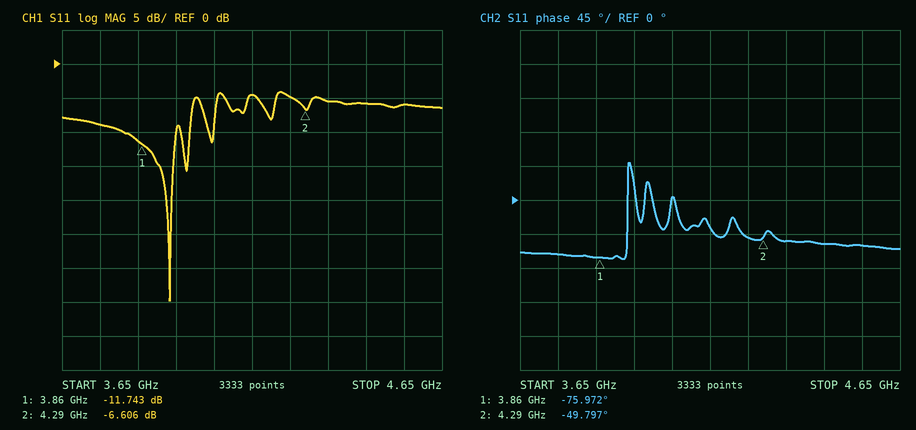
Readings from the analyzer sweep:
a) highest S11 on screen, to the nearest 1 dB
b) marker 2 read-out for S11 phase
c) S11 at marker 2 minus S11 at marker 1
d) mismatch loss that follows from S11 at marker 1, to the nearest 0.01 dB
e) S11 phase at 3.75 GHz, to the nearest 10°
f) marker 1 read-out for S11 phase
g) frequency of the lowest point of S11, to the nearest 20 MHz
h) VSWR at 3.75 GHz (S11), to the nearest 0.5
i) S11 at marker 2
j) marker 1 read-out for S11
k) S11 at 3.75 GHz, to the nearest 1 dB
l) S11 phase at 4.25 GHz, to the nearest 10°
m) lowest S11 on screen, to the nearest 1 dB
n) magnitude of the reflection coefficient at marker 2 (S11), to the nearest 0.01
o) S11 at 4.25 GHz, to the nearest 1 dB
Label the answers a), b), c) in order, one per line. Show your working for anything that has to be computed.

a) -4 dB
b) -49.797°
c) -6.606 − (-11.743) = 5.137 dB
d) −10 log10(1 − 10^(-11.743/10)) ≈ 0.30 dB
e) -70°
f) -75.972°
g) 3.94 GHz
h) |Γ| = 10^(-9/20) = 0.3548; VSWR = (1 + 0.3548)/(1 − 0.3548) ≈ 2.10, so 2.0 to the nearest 0.5
i) -6.606 dB
j) -11.743 dB
k) -9 dB
l) -50°
m) -35 dB
n) 10^(-6.606/20) ≈ 0.47
o) -5 dB
